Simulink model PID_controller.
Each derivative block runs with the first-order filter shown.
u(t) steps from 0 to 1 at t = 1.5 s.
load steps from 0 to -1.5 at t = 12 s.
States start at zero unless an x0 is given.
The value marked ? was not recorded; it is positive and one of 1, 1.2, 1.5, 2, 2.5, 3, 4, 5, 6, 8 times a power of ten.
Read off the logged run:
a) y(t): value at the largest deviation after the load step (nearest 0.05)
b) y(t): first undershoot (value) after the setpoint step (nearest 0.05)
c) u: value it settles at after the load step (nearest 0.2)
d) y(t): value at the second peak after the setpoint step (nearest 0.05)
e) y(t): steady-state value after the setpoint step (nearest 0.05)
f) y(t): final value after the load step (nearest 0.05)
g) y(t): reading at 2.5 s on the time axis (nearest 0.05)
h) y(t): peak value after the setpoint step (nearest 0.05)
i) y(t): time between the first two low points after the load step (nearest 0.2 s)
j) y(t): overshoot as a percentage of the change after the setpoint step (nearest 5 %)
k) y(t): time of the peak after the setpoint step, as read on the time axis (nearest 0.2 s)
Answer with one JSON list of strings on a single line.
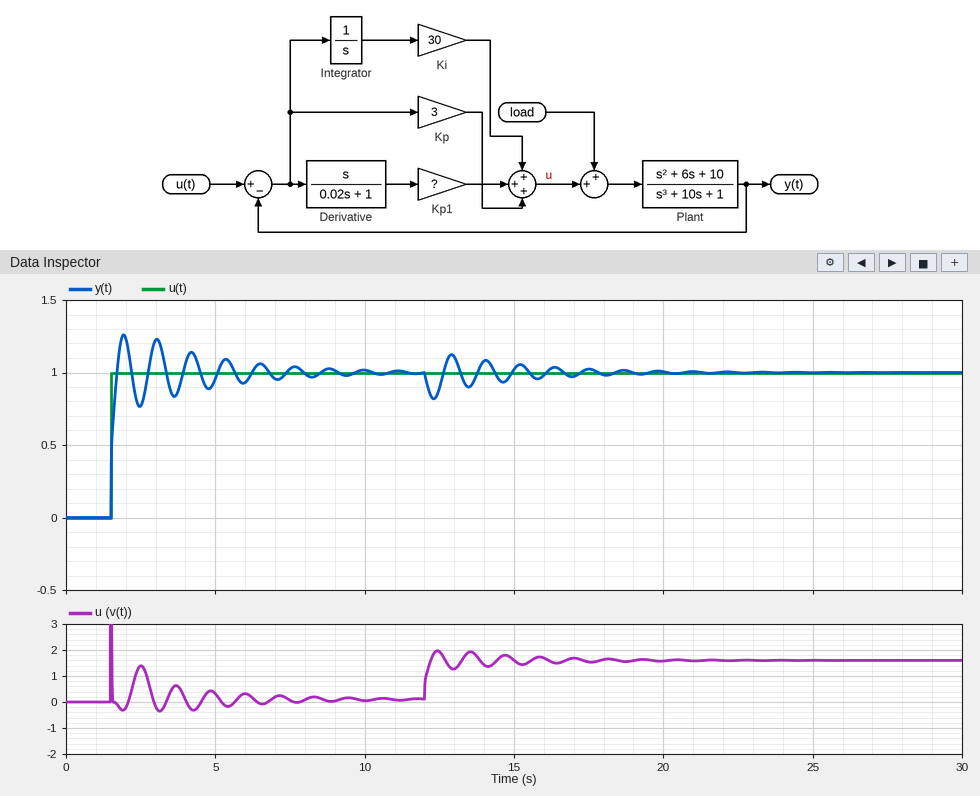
["0.80", "0.75", "1.6", "1.25", "1.00", "1.00", "0.75", "1.25", "1.2 s", "25 %", "2.0 s"]
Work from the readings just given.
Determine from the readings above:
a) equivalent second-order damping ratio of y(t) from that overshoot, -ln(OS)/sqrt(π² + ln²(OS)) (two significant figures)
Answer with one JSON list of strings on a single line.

["0.40"]
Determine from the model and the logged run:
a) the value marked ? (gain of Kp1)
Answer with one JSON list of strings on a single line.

["0.8"]
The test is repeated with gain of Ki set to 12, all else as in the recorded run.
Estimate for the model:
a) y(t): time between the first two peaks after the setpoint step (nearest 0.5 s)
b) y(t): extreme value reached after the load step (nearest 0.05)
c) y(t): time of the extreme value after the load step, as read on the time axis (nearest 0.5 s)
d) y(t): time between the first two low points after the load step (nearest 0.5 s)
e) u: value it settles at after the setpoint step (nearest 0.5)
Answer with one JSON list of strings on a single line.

["1.5 s", "0.75", "12.5 s", "1.5 s", "0.0"]
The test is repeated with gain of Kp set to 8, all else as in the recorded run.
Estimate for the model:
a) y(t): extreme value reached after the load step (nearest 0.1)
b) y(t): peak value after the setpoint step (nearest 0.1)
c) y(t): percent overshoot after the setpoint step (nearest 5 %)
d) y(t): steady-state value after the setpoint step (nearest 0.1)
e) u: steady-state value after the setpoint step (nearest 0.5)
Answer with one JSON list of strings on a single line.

["0.9", "1.2", "15 %", "1.0", "0.0"]
